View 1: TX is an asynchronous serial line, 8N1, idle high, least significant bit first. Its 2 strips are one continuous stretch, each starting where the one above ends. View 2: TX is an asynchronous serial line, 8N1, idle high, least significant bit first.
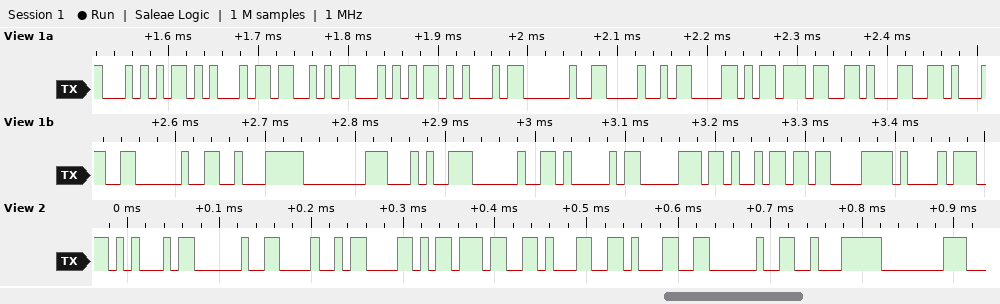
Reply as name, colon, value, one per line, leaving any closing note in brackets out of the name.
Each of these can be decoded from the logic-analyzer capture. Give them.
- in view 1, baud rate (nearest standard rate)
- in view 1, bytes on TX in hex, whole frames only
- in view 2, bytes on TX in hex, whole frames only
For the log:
in view 1, baud rate: 115200 baud
in view 1, bytes on TX in hex, whole frames only: 54 45 53 54 45 20 48 58 37 31 31 20 E2 80 94 20 41 70 69 C3 A1
in view 2, bytes on TX in hex, whole frames only: 45 20 48 58 37 31 31 20 E2 80
